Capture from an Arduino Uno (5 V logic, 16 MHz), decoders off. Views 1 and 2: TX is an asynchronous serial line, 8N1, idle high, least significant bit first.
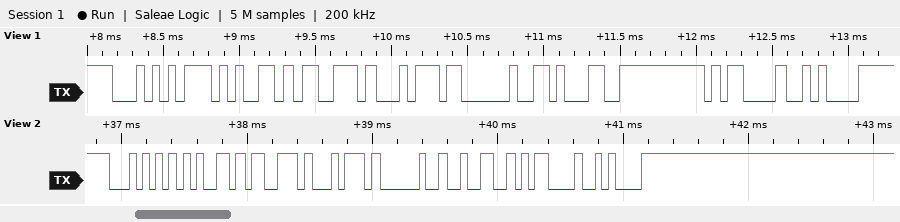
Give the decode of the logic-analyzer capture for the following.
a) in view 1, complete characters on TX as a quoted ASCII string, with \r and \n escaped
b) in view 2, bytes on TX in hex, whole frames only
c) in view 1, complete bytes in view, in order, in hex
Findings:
"Test 1\r\n"
0x54 0x65 0x73 0x74 0x20 0x32 0x0D 0x0A
0x54 0x65 0x73 0x74 0x20 0x31 0x0D 0x0A
